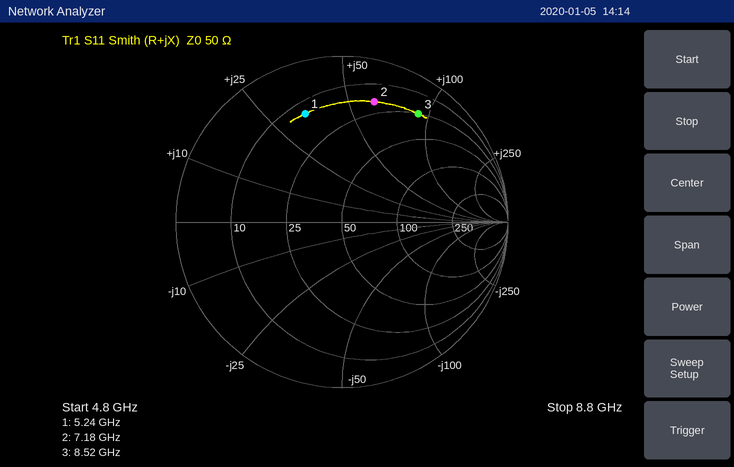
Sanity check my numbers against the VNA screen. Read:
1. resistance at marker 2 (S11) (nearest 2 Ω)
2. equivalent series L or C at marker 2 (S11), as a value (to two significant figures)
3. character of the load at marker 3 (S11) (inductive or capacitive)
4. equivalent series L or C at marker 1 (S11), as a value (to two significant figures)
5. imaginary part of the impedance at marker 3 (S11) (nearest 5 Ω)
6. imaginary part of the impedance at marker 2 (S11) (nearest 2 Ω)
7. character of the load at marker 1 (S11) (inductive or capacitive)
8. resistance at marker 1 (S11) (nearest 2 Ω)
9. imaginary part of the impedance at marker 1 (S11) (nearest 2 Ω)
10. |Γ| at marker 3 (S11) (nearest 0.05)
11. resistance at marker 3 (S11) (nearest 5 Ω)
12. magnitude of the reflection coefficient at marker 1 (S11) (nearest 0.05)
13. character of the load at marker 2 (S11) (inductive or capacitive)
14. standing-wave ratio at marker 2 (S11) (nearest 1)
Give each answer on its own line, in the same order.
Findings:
18 Ω
1.4 nH
inductive
1.0 nH
+90 Ω
+62 Ω
inductive
14 Ω
+34 Ω
0.80
25 Ω
0.70
inductive
7
